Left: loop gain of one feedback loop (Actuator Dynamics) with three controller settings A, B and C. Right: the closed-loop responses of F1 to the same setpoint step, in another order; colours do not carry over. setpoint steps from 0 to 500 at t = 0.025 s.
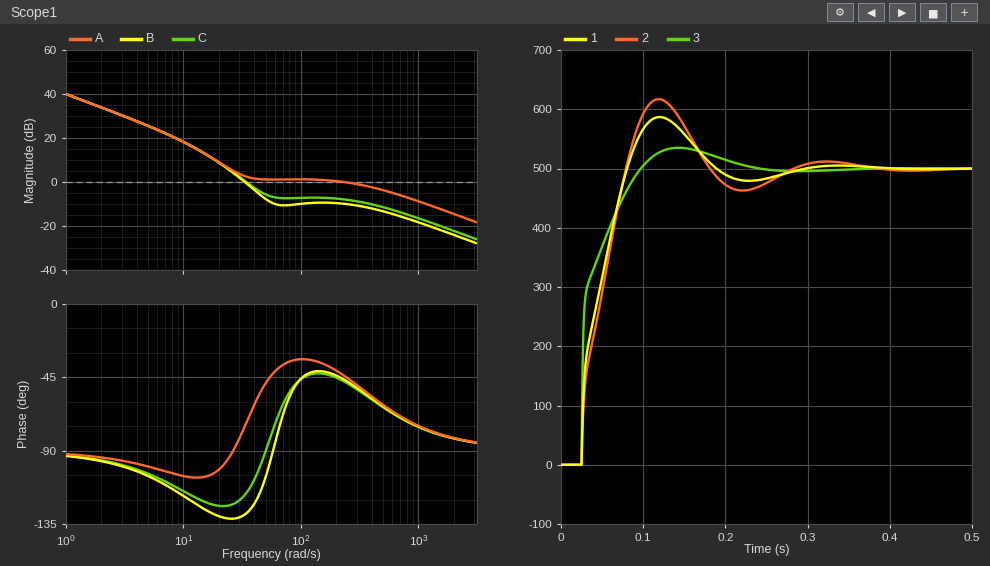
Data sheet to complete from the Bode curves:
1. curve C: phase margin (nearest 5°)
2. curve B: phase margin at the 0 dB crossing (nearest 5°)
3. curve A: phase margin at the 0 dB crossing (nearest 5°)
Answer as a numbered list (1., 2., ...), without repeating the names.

1. 65°
2. 50°
3. 135°
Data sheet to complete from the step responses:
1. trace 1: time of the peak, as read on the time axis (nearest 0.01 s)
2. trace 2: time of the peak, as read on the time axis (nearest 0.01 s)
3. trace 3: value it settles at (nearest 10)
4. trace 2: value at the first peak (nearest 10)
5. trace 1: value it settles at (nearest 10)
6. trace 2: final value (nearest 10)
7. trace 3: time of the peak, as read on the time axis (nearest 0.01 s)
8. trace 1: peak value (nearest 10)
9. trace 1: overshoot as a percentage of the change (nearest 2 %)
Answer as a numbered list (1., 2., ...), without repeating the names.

1. 0.12 s
2. 0.12 s
3. 500
4. 620
5. 500
6. 500
7. 0.14 s
8. 590
9. 18 %
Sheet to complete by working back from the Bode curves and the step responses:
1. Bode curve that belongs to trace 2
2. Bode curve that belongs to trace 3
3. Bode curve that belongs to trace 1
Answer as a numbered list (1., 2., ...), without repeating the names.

1. B
2. A
3. C
